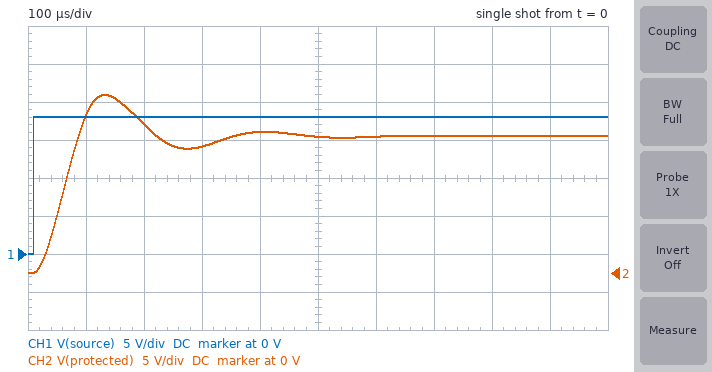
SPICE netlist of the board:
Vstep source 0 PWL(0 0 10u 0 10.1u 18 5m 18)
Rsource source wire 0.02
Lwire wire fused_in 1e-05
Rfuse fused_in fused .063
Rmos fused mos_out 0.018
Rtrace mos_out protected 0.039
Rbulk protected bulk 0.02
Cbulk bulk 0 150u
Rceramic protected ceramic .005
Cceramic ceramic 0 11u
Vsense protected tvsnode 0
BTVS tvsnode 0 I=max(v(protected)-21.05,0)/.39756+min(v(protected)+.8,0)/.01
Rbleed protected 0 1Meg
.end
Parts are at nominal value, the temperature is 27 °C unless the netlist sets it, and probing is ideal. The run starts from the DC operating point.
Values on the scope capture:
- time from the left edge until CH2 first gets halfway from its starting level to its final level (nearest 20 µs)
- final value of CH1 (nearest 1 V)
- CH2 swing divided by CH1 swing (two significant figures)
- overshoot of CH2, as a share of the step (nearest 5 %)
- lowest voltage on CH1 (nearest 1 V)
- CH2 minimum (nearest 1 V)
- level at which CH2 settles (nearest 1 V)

60 µs
18 V
1.3
30 %
0 V
0 V
18 V
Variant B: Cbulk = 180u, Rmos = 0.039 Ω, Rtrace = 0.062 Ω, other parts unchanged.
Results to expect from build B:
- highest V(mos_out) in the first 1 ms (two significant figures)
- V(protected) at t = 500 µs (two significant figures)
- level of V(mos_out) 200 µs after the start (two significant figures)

22 V
18 V
20 V
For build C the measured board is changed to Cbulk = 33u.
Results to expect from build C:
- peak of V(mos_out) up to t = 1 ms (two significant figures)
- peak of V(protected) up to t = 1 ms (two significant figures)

26 V
25 V
